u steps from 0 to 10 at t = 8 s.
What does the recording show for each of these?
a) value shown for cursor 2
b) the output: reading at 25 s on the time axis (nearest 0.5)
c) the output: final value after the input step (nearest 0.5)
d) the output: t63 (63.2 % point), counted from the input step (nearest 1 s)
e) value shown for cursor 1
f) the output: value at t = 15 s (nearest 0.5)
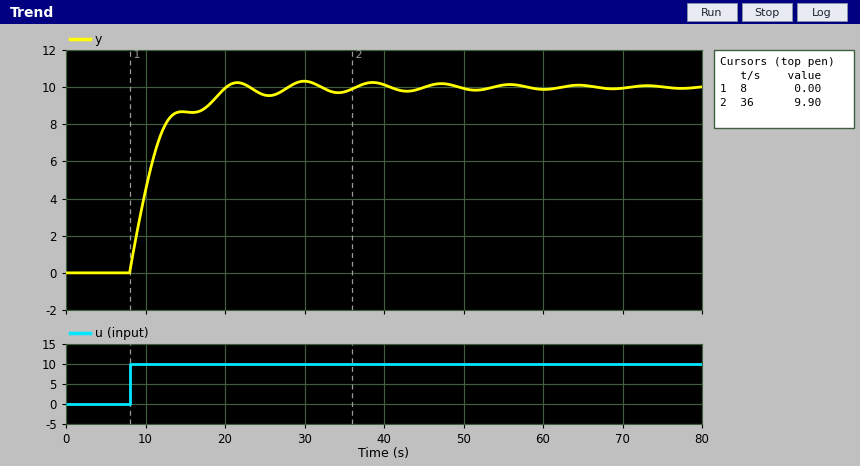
9.90
9.5
10.0
3 s
0.00
8.5
